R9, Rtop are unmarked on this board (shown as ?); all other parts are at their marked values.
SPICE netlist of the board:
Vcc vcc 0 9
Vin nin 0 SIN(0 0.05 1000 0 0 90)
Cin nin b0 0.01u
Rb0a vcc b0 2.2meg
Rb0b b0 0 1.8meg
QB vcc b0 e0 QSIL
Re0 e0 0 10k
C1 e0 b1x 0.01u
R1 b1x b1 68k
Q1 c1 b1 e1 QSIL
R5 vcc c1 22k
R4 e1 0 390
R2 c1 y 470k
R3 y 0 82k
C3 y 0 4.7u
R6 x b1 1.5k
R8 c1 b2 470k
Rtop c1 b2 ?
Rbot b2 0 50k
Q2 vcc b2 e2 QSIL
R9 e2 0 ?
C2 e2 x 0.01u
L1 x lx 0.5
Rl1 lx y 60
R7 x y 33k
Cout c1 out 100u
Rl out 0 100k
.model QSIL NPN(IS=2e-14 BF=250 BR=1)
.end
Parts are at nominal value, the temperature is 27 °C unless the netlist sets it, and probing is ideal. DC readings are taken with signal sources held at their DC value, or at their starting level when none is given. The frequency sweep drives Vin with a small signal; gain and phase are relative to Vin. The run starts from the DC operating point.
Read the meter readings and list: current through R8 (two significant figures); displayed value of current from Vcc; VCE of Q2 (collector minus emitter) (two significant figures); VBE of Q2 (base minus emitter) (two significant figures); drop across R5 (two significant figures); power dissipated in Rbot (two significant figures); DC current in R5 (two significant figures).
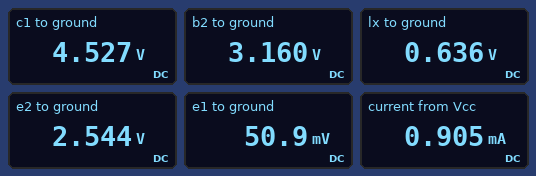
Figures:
2.9 µA
0.905 mA
6.5 V
620 mV
4.5 V
200 µW
200 µA
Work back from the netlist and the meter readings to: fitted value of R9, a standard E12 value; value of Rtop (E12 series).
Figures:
5.6 kΩ
22 kΩ
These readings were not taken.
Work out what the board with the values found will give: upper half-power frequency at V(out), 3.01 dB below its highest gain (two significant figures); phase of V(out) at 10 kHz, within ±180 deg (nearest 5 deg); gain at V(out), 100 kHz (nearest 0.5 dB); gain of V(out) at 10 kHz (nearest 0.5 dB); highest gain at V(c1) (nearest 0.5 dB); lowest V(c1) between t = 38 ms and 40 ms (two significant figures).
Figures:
590 Hz
135 deg
-30.0 dB
-27.0 dB
14.5 dB
4.5 V
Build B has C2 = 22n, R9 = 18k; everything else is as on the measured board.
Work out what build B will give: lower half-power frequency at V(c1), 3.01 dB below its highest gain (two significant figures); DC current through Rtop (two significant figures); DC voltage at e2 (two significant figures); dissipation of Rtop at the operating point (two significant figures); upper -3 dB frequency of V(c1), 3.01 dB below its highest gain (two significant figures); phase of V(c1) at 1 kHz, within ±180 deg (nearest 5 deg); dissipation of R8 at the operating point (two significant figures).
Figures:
360 Hz
61 µA
2.6 V
83 µW
400 Hz
95 deg
3.9 µW
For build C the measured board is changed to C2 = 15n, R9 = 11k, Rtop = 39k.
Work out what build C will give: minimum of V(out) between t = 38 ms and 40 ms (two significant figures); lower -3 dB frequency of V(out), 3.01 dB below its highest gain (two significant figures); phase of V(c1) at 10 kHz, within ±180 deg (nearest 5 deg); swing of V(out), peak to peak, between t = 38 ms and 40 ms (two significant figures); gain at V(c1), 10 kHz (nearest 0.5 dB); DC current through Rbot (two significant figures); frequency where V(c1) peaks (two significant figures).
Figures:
-18 mV
460 Hz
150 deg
35 mV
-26.5 dB
53 µA
490 Hz
